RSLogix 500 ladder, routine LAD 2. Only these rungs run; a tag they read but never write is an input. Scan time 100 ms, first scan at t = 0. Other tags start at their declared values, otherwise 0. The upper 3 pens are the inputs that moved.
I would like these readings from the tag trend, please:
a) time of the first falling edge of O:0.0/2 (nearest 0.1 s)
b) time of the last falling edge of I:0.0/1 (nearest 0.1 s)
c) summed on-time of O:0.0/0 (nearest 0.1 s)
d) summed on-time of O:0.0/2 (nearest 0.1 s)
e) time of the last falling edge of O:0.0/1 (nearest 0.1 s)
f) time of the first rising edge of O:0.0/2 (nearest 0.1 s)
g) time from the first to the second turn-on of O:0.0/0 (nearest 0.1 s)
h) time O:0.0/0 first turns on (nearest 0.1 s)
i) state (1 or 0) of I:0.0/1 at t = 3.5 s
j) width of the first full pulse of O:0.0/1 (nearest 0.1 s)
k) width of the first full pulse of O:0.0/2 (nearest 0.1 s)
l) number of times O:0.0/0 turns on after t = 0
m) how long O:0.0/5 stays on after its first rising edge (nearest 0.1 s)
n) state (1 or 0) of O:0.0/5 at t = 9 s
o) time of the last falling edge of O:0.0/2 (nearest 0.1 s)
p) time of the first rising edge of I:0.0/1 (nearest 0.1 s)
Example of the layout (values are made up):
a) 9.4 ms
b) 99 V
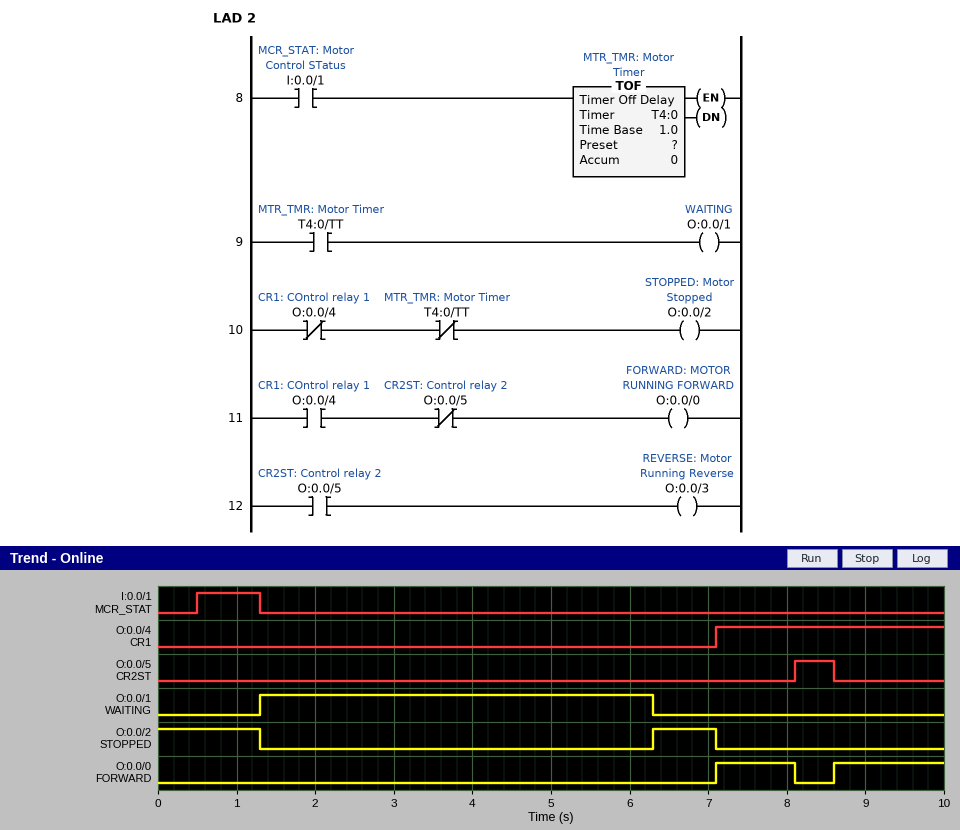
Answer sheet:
a) 1.3 s
b) 1.3 s
c) 2.4 s
d) 2.1 s
e) 6.3 s
f) 6.3 s
g) 1.5 s
h) 7.1 s
i) 0
j) 5.0 s
k) 0.8 s
l) 2
m) 0.5 s
n) 0
o) 7.1 s
p) 0.5 s
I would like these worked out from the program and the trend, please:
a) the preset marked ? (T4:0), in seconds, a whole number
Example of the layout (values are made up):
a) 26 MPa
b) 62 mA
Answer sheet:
a) 5 s
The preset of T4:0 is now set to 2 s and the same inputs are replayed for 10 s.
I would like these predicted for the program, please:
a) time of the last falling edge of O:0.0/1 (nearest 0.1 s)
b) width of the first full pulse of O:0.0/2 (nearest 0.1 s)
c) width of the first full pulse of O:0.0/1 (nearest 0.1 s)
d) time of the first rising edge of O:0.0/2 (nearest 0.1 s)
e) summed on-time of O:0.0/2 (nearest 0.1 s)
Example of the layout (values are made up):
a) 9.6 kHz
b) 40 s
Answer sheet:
a) 3.3 s
b) 3.8 s
c) 2.0 s
d) 3.3 s
e) 5.1 s
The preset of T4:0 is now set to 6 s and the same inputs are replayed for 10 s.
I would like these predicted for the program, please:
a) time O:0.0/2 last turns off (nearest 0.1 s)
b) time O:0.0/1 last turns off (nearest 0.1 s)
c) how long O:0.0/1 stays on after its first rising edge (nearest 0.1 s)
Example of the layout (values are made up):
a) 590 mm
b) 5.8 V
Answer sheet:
a) 1.3 s
b) 7.3 s
c) 6.0 s
